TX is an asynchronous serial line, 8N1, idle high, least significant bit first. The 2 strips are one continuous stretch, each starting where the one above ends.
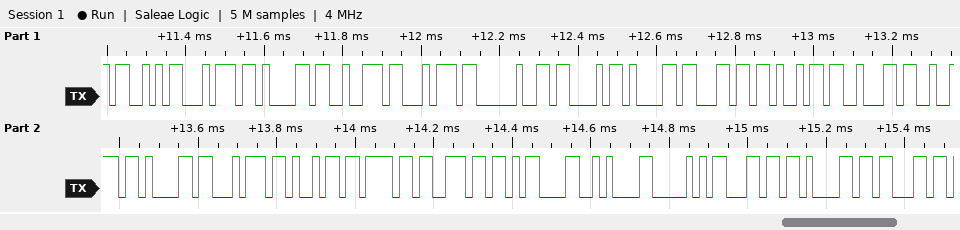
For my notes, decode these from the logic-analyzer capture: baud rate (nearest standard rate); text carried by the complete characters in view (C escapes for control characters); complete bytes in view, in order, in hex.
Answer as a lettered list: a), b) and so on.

a) 57600 baud
b) "Start Calibration\r\nPlac"
c) 53 74 61 72 74 20 43 61 6C 69 62 72 61 74 69 6F 6E 0D 0A 50 6C 61 63
